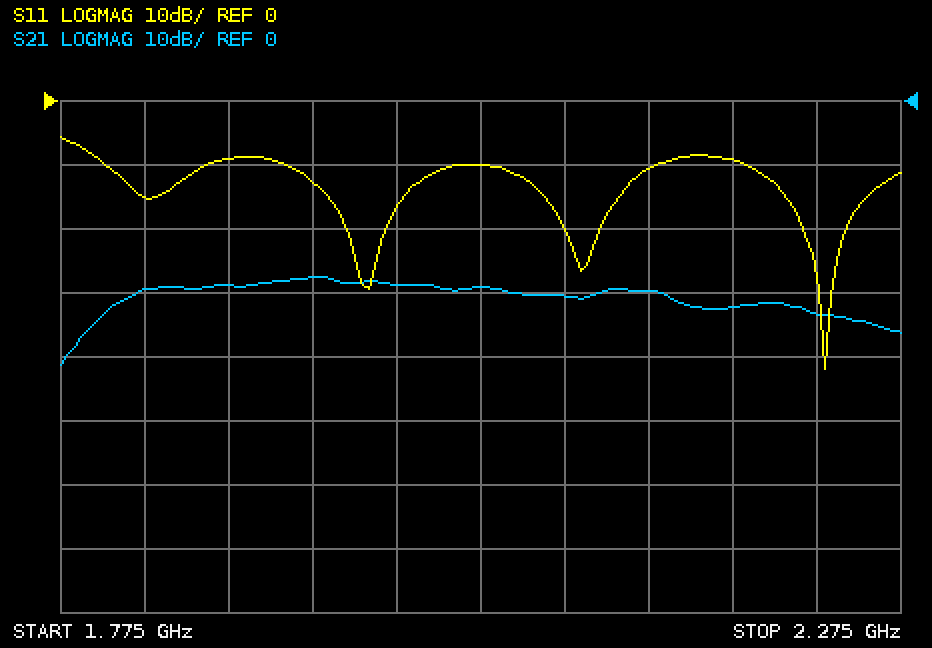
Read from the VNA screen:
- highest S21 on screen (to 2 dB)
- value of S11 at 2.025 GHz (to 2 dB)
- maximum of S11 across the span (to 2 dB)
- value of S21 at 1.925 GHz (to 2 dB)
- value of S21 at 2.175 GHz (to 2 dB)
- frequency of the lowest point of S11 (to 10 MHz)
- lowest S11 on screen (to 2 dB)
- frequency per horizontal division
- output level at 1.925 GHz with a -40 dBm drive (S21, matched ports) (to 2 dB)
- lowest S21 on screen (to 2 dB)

-28 dB
-10 dB
-6 dB
-28 dB
-32 dB
2.23 GHz
-42 dB
50 MHz
-68 dBm
-42 dB
